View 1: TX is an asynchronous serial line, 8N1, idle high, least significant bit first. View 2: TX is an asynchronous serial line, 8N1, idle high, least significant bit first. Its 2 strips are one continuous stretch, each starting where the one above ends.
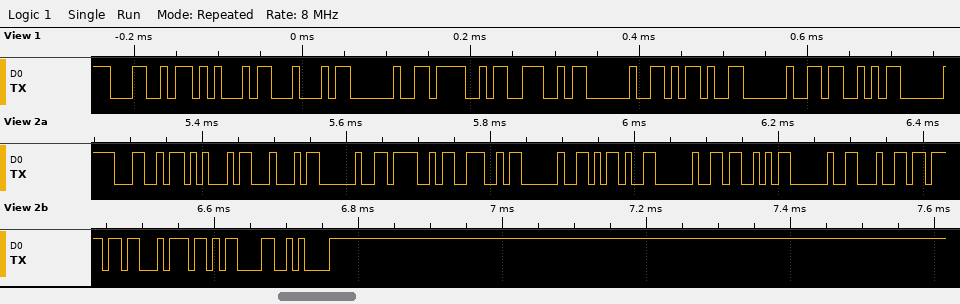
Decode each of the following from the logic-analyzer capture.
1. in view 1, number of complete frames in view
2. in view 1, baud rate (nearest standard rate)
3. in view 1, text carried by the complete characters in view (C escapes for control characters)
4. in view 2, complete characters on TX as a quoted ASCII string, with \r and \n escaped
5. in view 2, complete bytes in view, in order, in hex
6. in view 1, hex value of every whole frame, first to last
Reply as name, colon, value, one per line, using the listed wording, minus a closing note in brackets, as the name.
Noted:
in view 1, number of complete frames in view: 10
in view 1, baud rate: 115200 baud
in view 1, text carried by the complete characters in view: "LED ON - S"
in view 2, complete characters on TX as a quoted ASCII string, with \r and \n escaped: "LED ON - S dot\r\n"
in view 2, complete bytes in view, in order, in hex: 4C 45 44 20 4F 4E 20 2D 20 53 20 64 6F 74 0D 0A
in view 1, hex value of every whole frame, first to last: 0x4C 0x45 0x44 0x20 0x4F 0x4E 0x20 0x2D 0x20 0x53
